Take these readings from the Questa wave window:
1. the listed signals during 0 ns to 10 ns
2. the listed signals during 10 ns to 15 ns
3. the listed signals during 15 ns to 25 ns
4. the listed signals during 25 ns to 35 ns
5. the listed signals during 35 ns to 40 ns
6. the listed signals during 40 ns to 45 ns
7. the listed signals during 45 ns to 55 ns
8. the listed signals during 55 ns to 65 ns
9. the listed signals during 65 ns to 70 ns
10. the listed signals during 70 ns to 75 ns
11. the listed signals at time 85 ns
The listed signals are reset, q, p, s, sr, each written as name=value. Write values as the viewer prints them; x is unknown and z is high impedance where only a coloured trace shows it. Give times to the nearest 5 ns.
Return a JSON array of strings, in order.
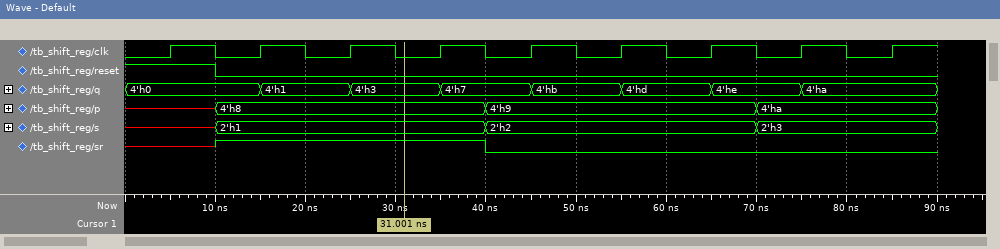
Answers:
["reset=1, q=4'h0, p=x, s=x, sr=x", "reset=0, q=4'h0, p=4'h8, s=2'h1, sr=1", "reset=0, q=4'h1, p=4'h8, s=2'h1, sr=1", "reset=0, q=4'h3, p=4'h8, s=2'h1, sr=1", "reset=0, q=4'h7, p=4'h8, s=2'h1, sr=1", "reset=0, q=4'h7, p=4'h9, s=2'h2, sr=0", "reset=0, q=4'hb, p=4'h9, s=2'h2, sr=0", "reset=0, q=4'hd, p=4'h9, s=2'h2, sr=0", "reset=0, q=4'he, p=4'h9, s=2'h2, sr=0", "reset=0, q=4'he, p=4'ha, s=2'h3, sr=0", "reset=0, q=4'ha, p=4'ha, s=2'h3, sr=0"]
